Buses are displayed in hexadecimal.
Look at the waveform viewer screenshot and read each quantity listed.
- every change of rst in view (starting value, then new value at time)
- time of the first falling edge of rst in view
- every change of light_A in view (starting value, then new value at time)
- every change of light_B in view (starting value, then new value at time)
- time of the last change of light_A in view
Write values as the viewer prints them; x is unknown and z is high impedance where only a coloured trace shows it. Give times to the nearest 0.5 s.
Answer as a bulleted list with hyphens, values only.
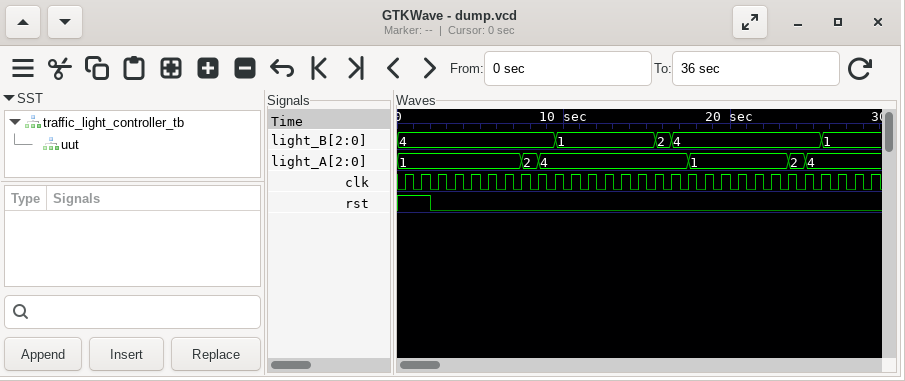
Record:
- 1, 0 at 2 s
- 2 s
- 1, 2 at 7.5 s, 4 at 8.5 s, 1 at 17.5 s, 2 at 23.5 s, 4 at 24.5 s
- 4, 1 at 9.5 s, 2 at 15.5 s, 4 at 16.5 s, 1 at 25.5 s
- 24.5 s
